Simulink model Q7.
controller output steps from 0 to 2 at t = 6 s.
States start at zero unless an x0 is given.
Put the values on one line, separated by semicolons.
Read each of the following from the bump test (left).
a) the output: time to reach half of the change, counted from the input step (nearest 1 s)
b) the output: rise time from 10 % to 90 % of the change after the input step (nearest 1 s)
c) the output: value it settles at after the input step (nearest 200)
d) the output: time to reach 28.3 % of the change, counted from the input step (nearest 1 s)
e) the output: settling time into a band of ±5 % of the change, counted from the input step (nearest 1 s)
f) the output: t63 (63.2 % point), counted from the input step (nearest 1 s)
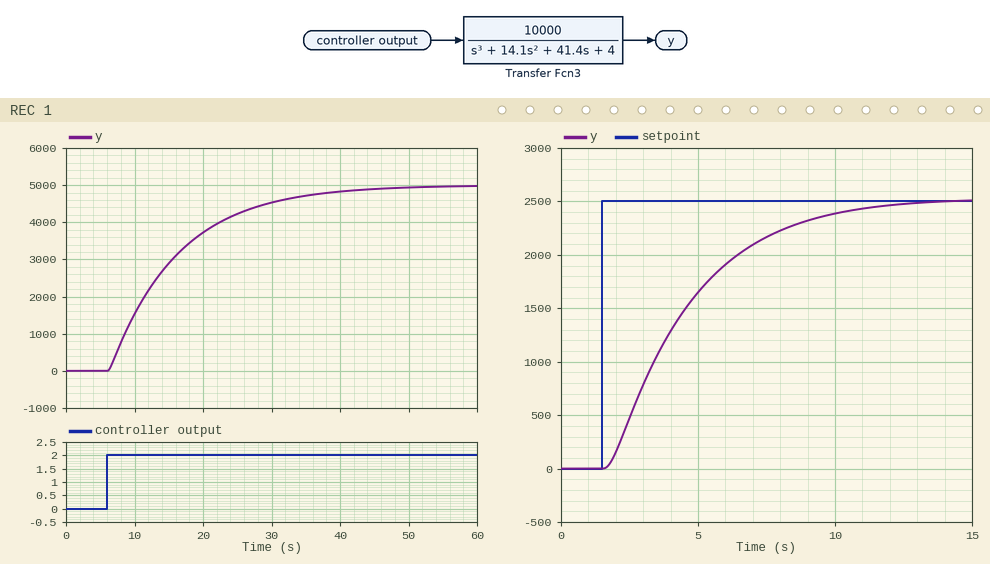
7 s; 22 s; 5000; 4 s; 30 s; 10 s
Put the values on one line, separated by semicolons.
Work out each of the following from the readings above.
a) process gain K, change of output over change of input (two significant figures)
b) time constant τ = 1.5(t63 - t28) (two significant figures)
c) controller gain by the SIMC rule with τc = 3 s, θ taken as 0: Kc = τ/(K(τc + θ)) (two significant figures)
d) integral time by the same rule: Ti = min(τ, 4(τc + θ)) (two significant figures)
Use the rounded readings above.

2500; 9.0 s; 0.0012; 9.0 s
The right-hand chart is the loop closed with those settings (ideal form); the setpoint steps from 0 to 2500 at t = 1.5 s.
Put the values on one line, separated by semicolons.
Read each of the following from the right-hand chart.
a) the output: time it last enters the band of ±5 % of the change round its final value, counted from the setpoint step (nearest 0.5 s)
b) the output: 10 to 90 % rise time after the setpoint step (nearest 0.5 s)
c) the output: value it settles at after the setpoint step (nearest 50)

8.5 s; 6.0 s; 2500
